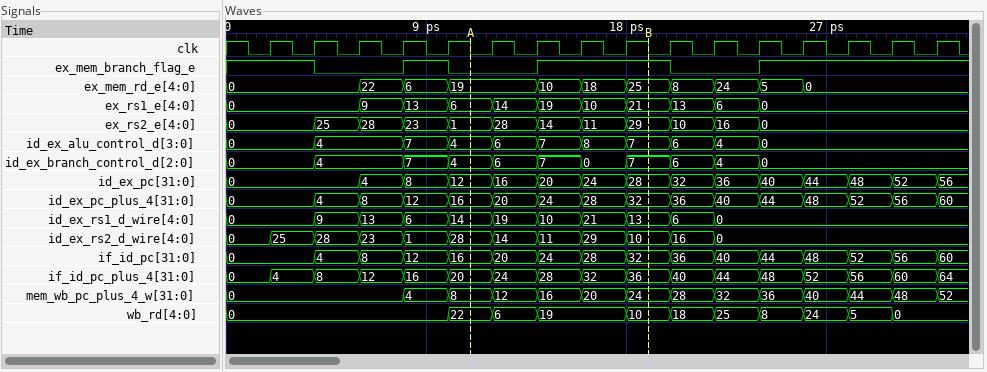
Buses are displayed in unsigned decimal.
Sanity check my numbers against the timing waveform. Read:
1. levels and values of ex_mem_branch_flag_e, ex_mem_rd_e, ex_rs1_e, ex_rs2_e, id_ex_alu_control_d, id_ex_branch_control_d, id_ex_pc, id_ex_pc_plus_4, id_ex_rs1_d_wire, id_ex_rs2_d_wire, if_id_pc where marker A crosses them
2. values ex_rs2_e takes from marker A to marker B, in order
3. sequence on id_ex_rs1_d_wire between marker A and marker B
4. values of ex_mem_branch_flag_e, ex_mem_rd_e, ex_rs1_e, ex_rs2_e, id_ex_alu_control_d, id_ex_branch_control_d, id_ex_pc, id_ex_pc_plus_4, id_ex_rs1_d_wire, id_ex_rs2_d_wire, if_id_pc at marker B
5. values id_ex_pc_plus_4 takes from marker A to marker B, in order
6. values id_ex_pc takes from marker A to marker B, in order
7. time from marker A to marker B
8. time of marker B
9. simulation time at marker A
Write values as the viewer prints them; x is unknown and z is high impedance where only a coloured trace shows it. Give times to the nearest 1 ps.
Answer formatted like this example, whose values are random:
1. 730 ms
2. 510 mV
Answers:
1. ex_mem_branch_flag_e=0, ex_mem_rd_e=19, ex_rs1_e=6, ex_rs2_e=1, id_ex_alu_control_d=4, id_ex_branch_control_d=4, id_ex_pc=12, id_ex_pc_plus_4=16, id_ex_rs1_d_wire=14, id_ex_rs2_d_wire=28, if_id_pc=16
2. 1, 28, 14, 11, 29
3. 14, 19, 10, 21, 13
4. ex_mem_branch_flag_e=1, ex_mem_rd_e=25, ex_rs1_e=21, ex_rs2_e=29, id_ex_alu_control_d=7, id_ex_branch_control_d=7, id_ex_pc=28, id_ex_pc_plus_4=32, id_ex_rs1_d_wire=13, id_ex_rs2_d_wire=10, if_id_pc=32
5. 16, 20, 24, 28, 32
6. 12, 16, 20, 24, 28
7. 8 ps
8. 19 ps
9. 11 ps
